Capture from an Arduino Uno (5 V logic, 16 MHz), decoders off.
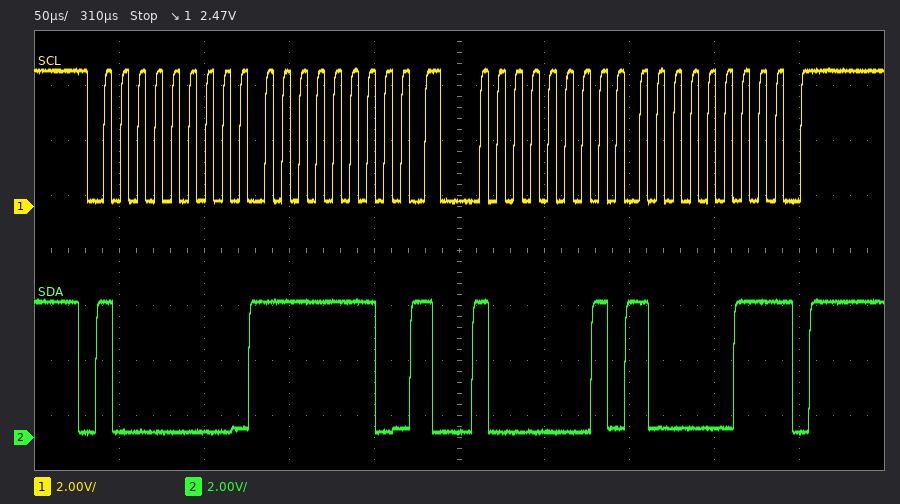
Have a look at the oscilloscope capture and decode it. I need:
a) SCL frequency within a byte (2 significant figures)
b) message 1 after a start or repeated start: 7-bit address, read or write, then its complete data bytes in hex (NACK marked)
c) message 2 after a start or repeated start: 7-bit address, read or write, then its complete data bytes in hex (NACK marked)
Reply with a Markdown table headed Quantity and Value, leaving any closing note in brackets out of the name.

| Quantity | Value |
|---|---|
| SCL frequency within a byte | 100 kHz |
| message 1 after a start or repeated start: 7-bit address, read or write, then its complete data bytes in hex | 0x40 write: FE |
| message 2 after a start or repeated start: 7-bit address, read or write, then its complete data bytes in hex | 0x40 read: 83 NACK |
